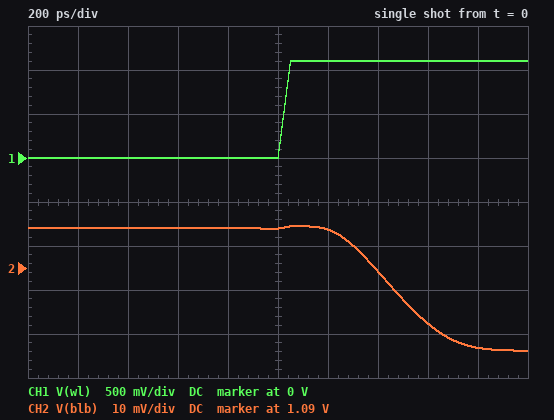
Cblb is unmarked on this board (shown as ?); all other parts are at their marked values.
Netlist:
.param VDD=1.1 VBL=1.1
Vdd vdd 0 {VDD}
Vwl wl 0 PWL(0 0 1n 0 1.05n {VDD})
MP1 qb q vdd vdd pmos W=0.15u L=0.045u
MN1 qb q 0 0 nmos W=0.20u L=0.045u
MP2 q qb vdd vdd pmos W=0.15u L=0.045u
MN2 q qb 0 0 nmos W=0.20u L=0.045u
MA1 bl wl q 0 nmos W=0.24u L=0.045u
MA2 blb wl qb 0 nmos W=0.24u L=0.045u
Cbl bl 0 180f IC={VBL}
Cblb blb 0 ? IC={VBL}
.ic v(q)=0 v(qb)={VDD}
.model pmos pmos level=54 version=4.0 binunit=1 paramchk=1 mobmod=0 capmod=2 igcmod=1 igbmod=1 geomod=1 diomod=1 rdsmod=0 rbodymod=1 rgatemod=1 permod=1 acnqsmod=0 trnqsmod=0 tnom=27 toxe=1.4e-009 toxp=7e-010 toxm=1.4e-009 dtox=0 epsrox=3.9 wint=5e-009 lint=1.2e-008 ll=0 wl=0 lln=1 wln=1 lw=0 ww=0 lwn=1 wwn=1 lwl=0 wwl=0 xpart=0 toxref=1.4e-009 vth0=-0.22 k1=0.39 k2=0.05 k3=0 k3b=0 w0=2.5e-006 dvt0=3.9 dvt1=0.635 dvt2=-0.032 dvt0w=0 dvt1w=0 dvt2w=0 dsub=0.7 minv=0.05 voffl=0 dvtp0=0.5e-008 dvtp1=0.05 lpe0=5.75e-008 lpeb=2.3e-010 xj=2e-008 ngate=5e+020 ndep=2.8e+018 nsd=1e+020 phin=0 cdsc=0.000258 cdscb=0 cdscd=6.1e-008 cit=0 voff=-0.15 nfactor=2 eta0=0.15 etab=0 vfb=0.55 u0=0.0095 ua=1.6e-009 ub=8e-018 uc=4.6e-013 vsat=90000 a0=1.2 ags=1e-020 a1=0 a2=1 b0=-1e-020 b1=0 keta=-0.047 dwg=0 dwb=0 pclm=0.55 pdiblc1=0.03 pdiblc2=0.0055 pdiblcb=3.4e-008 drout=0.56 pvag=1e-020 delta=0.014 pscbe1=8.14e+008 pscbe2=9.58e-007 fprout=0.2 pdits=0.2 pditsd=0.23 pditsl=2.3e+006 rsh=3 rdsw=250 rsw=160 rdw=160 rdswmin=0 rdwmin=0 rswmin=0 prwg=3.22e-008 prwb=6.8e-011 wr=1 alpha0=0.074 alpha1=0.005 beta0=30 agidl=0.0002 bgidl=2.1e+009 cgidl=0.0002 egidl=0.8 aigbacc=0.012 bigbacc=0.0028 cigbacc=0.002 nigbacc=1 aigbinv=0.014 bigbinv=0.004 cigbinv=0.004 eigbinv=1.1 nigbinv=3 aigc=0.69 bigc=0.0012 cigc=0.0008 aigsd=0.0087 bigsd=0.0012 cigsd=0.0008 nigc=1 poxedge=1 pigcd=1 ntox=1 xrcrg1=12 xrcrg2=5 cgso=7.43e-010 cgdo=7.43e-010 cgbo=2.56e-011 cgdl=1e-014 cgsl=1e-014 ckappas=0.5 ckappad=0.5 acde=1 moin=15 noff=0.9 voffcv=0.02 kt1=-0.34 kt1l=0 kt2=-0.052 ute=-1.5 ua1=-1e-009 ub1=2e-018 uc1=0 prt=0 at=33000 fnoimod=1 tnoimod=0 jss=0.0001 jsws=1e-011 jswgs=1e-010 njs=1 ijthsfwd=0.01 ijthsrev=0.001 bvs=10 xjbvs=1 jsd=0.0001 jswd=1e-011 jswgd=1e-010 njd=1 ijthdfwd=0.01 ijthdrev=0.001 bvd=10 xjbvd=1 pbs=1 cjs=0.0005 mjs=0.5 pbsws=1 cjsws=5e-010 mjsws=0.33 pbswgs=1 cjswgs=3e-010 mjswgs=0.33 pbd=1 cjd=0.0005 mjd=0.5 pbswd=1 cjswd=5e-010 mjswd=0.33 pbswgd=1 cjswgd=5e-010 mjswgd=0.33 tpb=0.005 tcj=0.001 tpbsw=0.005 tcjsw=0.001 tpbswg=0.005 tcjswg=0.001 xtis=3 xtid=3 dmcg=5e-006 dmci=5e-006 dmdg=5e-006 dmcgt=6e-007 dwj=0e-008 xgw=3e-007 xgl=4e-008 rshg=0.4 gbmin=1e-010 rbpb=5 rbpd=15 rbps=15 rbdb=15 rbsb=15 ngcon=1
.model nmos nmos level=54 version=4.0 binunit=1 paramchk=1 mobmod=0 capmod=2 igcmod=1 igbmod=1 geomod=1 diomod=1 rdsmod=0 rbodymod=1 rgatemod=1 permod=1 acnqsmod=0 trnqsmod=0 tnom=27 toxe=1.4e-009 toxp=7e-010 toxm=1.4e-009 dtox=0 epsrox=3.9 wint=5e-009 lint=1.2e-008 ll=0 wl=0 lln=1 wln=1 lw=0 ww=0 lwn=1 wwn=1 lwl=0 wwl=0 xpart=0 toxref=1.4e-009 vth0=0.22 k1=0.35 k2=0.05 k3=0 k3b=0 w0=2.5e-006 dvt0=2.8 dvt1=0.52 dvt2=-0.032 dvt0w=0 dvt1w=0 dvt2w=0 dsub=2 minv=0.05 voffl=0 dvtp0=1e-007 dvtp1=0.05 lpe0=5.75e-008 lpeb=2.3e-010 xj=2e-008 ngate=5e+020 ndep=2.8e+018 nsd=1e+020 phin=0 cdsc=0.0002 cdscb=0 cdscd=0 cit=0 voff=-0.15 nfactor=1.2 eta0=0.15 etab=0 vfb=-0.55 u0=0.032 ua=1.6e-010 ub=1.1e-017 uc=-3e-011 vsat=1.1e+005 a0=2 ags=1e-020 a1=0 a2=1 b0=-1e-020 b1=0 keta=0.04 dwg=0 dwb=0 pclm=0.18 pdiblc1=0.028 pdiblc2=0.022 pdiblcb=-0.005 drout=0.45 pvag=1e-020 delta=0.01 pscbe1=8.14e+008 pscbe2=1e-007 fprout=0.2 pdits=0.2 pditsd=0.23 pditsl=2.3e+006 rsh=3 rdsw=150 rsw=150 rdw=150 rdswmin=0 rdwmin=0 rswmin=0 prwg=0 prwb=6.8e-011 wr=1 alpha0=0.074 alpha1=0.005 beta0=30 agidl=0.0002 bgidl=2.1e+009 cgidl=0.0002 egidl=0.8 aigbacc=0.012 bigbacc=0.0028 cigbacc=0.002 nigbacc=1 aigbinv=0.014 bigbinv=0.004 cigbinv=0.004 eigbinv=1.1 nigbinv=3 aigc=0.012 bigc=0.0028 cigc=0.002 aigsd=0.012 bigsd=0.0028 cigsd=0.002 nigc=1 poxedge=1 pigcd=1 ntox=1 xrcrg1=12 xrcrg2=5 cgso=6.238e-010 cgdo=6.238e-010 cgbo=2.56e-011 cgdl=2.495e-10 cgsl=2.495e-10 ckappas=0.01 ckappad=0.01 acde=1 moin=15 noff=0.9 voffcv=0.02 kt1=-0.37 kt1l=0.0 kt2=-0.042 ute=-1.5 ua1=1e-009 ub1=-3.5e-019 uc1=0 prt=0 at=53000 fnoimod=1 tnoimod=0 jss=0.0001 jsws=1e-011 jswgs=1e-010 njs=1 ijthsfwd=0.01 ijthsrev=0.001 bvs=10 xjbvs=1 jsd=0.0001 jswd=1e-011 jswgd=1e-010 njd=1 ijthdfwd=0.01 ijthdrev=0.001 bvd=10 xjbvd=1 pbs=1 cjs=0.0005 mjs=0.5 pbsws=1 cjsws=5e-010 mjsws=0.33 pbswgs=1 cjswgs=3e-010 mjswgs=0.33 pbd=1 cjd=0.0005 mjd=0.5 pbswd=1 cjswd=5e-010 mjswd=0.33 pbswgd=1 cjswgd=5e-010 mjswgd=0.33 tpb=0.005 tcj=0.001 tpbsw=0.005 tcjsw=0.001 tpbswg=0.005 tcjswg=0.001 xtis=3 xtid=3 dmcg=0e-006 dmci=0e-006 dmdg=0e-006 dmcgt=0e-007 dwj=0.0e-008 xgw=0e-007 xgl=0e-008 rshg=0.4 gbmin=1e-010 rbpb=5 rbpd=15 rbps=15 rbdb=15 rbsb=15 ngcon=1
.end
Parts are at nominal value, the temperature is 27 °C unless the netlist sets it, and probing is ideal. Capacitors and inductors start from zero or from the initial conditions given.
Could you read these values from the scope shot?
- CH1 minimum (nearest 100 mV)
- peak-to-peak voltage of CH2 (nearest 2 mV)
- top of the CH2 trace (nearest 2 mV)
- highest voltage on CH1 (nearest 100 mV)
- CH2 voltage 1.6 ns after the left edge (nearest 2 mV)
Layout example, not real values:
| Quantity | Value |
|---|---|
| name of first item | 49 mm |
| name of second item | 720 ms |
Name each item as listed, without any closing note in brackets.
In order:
| Quantity | Value |
|---|---|
| CH1 minimum | 0 V |
| peak-to-peak voltage of CH2 | 28 mV |
| top of the CH2 trace | 1.100 V |
| highest voltage on CH1 | 1.1 V |
| CH2 voltage 1.6 ns after the left edge | 1.078 V |
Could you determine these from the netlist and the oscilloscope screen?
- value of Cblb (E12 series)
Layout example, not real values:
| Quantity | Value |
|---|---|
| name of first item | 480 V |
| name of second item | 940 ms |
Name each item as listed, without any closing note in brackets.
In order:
| Quantity | Value |
|---|---|
| value of Cblb | 390 fF |
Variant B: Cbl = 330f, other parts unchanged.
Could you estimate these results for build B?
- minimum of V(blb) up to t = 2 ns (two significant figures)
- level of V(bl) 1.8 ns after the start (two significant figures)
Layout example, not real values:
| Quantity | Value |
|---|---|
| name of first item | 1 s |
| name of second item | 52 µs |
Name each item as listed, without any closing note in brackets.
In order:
| Quantity | Value |
|---|---|
| minimum of V(blb) up to t = 2 ns | 1.0 V |
| level of V(bl) 1.8 ns after the start | 880 mV |
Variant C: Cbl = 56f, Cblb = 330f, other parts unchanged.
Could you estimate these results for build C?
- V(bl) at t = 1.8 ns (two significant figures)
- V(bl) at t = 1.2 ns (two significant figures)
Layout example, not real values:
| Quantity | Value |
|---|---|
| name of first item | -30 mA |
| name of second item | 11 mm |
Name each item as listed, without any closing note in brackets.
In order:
| Quantity | Value |
|---|---|
| V(bl) at t = 1.8 ns | 63 mV |
| V(bl) at t = 1.2 ns | 700 mV |
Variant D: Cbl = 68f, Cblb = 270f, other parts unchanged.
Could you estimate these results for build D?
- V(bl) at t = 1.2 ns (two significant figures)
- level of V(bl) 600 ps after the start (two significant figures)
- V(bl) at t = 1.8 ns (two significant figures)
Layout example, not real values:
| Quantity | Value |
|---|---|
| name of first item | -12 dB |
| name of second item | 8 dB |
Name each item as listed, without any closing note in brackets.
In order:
| Quantity | Value |
|---|---|
| V(bl) at t = 1.2 ns | 770 mV |
| level of V(bl) 600 ps after the start | 1.1 V |
| V(bl) at t = 1.8 ns | 120 mV |
